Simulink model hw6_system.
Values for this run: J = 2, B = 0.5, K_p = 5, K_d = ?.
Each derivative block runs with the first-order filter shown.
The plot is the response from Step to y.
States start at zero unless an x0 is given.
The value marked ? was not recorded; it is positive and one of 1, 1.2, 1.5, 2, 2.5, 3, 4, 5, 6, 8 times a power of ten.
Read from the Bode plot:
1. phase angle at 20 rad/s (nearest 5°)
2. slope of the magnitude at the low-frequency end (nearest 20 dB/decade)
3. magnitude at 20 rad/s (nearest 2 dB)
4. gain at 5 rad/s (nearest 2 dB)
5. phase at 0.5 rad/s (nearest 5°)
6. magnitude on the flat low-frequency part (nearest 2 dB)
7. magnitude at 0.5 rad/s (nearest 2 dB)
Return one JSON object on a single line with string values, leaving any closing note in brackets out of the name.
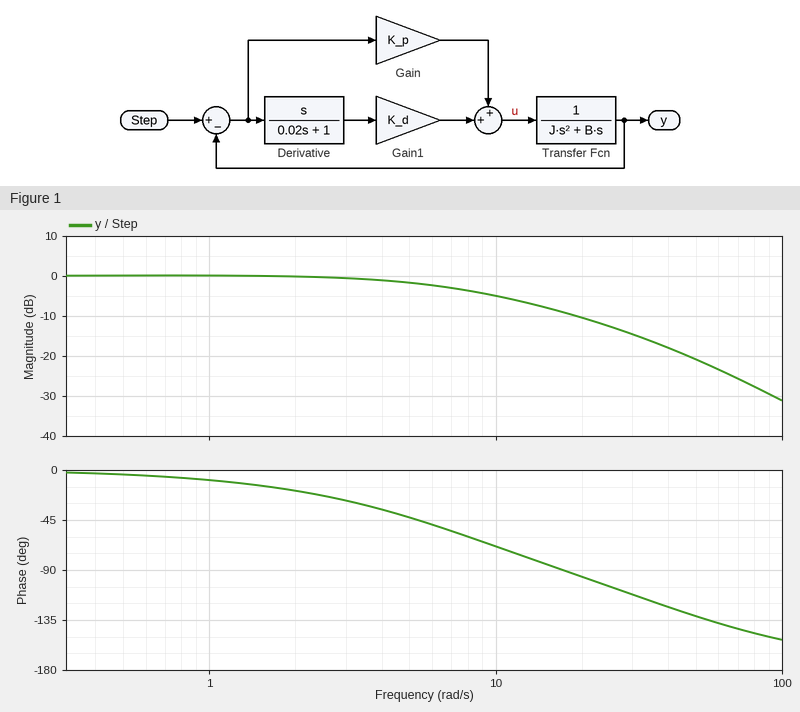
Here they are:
{"phase angle at 20 rad/s": "-95°", "slope of the magnitude at the low-frequency end": "0 dB/decade", "magnitude at 20 rad/s": "-10 dB", "gain at 5 rad/s": "-2 dB", "phase at 0.5 rad/s": "-5°", "magnitude on the flat low-frequency part": "0 dB", "magnitude at 0.5 rad/s": "0 dB"}
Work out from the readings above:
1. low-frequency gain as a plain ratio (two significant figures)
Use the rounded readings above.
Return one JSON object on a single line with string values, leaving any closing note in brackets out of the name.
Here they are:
{"low-frequency gain as a plain ratio": "1.0"}
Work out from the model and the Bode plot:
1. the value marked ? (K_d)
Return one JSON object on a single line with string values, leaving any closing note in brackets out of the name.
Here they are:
{"the value marked ?": "12"}
